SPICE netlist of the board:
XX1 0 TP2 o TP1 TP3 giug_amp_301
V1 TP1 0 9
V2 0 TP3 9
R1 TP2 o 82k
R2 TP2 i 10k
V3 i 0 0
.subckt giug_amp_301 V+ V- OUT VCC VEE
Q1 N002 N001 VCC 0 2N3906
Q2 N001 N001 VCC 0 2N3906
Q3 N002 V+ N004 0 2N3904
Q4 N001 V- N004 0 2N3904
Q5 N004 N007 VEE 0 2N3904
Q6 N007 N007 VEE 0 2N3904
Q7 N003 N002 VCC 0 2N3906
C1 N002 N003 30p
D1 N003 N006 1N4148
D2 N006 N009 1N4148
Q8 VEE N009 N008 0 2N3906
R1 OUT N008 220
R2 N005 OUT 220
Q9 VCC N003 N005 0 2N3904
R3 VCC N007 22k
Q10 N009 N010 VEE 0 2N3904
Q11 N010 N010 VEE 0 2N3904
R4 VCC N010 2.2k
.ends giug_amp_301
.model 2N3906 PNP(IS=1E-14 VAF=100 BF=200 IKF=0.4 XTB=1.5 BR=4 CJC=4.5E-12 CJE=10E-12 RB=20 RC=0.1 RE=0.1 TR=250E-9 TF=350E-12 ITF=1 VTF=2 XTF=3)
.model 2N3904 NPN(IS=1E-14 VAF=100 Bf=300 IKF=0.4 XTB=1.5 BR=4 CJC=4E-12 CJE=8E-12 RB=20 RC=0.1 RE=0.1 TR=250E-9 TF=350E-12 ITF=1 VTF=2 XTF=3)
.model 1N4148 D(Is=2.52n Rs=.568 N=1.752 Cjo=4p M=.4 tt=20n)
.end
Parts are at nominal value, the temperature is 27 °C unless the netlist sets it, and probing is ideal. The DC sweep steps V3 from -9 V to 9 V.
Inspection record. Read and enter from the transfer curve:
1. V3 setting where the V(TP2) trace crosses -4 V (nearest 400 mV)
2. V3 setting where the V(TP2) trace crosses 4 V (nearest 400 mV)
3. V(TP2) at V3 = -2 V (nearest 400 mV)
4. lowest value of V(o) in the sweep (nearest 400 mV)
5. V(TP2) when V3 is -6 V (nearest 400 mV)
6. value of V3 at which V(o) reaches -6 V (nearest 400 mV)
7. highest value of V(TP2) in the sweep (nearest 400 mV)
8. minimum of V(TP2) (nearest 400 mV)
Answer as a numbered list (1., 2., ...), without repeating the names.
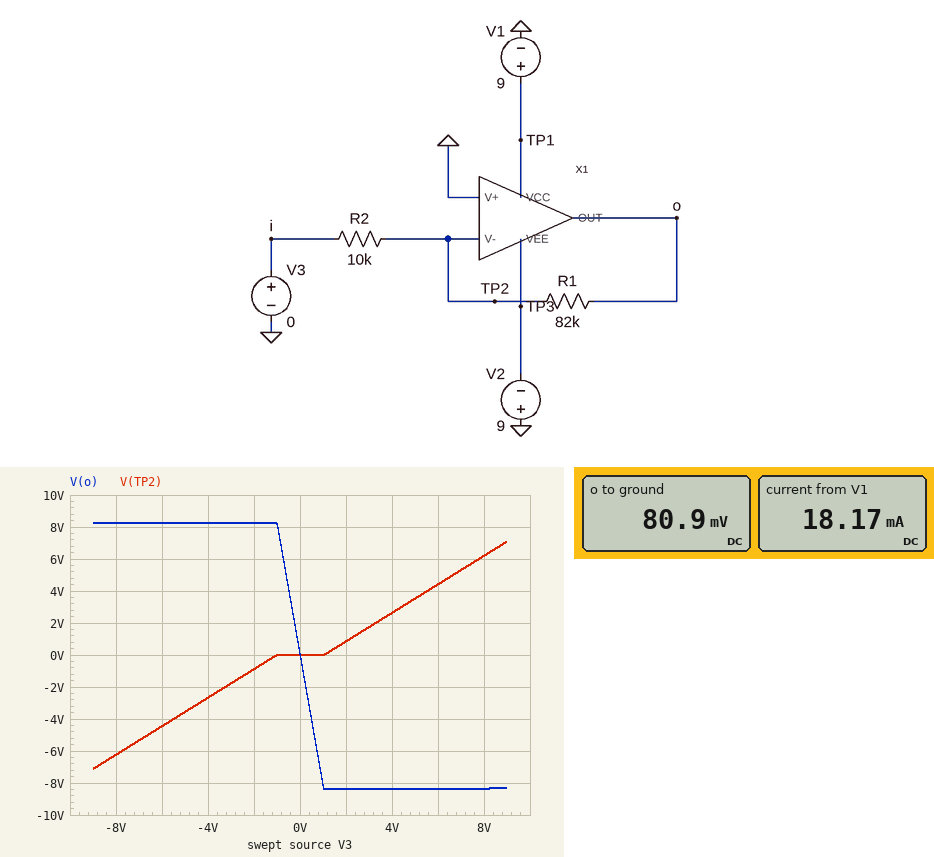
1. -5.6 V
2. 5.6 V
3. -800 mV
4. -8.4 V
5. -4.4 V
6. 800 mV
7. 7.2 V
8. -7.2 V
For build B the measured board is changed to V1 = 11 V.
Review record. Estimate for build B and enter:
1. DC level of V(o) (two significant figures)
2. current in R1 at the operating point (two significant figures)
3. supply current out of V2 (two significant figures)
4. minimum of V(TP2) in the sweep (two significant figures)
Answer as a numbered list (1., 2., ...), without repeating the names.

1. 91 mV
2. 1.1 µA
3. 20 mA
4. -6.9 V
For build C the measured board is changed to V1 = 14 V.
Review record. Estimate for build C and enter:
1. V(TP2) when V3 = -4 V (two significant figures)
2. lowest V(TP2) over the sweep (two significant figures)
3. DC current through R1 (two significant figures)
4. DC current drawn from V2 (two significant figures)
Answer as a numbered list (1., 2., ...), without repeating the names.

1. -2.1 V
2. -6.6 V
3. 1.3 µA
4. 23 mA
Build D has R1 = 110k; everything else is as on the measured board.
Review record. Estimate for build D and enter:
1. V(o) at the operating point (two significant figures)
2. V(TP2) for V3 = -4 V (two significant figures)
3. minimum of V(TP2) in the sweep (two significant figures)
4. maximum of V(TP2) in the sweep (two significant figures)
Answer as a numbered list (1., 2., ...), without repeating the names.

1. 110 mV
2. -3.0 V
3. -7.6 V
4. 7.5 V
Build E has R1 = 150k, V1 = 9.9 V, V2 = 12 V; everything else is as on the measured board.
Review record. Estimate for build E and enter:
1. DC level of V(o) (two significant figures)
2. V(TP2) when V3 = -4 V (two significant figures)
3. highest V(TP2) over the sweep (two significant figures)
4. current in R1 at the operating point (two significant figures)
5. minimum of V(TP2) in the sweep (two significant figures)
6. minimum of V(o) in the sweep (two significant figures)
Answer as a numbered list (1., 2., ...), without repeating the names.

1. 200 mV
2. -3.2 V
3. 7.7 V
4. 1.3 µA
5. -7.9 V
6. -11 V
